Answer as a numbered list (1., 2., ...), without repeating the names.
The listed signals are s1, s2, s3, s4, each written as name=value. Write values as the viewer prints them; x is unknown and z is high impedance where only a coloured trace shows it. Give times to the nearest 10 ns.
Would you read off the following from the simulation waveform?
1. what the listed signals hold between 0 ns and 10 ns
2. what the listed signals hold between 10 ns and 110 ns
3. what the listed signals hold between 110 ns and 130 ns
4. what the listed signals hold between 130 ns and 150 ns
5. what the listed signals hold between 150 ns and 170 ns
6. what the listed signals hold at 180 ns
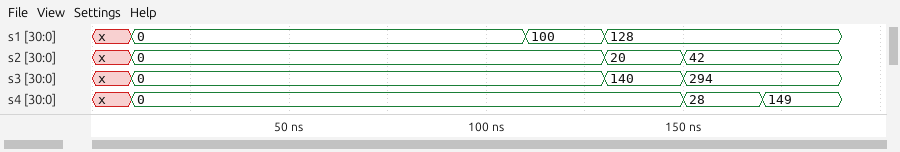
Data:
1. s1=x, s2=x, s3=x, s4=x
2. s1=0, s2=0, s3=0, s4=0
3. s1=100, s2=0, s3=0, s4=0
4. s1=128, s2=20, s3=140, s4=0
5. s1=128, s2=42, s3=294, s4=28
6. s1=128, s2=42, s3=294, s4=149
